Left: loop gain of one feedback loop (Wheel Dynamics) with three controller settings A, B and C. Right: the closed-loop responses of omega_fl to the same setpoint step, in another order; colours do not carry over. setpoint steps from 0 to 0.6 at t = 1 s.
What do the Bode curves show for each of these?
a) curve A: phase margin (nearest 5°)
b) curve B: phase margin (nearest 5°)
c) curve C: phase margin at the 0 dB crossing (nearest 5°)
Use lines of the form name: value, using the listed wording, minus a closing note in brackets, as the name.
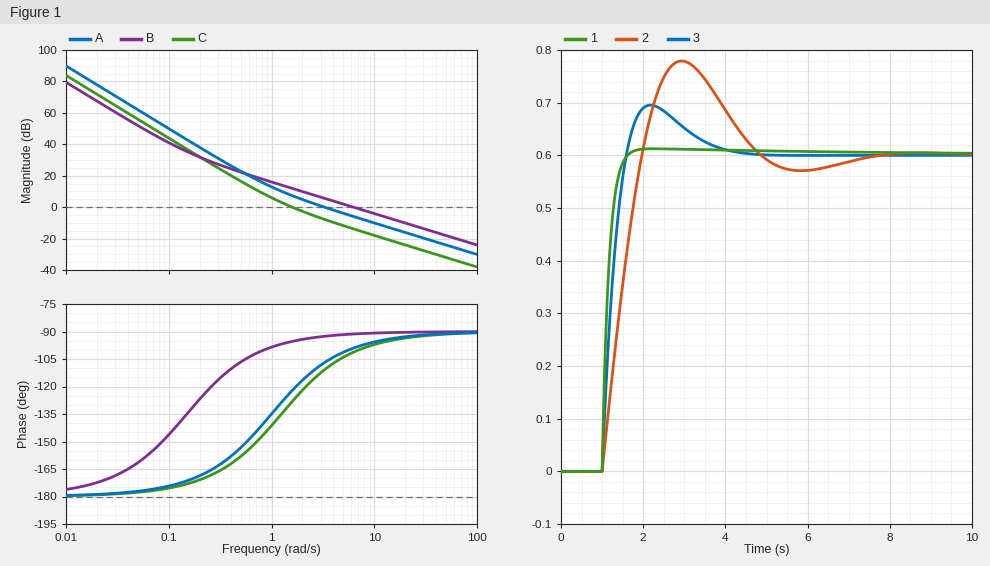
curve A: phase margin: 75°
curve B: phase margin: 90°
curve C: phase margin at the 0 dB crossing: 50°
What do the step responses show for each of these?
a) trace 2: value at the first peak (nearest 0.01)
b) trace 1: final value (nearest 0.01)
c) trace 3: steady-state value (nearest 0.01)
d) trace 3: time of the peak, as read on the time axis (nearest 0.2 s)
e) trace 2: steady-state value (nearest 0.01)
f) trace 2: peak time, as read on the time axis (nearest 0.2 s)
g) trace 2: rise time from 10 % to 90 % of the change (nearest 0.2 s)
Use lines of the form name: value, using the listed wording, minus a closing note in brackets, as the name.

trace 2: value at the first peak: 0.78
trace 1: final value: 0.60
trace 3: steady-state value: 0.60
trace 3: time of the peak, as read on the time axis: 2.2 s
trace 2: steady-state value: 0.60
trace 2: peak time, as read on the time axis: 3.0 s
trace 2: rise time from 10 % to 90 % of the change: 0.8 s
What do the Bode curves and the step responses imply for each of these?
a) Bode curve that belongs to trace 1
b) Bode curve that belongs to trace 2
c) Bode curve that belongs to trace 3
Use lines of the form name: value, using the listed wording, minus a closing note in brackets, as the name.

Bode curve that belongs to trace 1: B
Bode curve that belongs to trace 2: C
Bode curve that belongs to trace 3: A
